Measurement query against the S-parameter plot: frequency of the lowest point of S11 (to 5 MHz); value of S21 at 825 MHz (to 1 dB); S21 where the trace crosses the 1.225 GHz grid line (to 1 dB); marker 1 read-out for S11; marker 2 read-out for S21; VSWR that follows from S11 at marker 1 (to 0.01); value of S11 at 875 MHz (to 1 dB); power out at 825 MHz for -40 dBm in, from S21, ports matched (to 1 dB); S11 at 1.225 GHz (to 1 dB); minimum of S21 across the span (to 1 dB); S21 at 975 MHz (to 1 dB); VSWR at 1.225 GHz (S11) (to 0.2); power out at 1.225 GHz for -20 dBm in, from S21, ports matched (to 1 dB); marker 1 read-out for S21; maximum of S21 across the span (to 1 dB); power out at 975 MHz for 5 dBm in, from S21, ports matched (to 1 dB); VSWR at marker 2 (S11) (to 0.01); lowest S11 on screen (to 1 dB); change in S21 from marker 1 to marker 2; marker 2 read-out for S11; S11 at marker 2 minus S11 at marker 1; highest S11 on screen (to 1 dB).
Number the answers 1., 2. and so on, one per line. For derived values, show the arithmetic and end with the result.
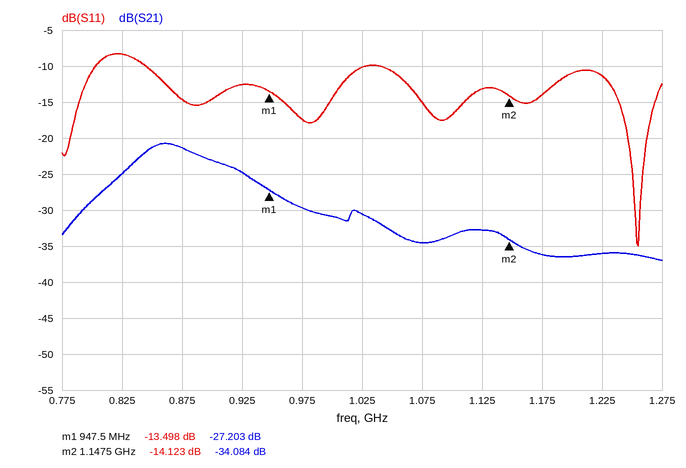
1. 1.255 GHz
2. -25 dB
3. -36 dB
4. -13.498 dB
5. -34.084 dB
6. (1 + 0.2114)/(1 − 0.2114) ≈ 1.54
7. -15 dB
8. -40 dBm + (-25 dB) = -65 dBm
9. -11 dB
10. -37 dB
11. -30 dB
12. |Γ| = 10^(-11/20) = 0.2818; VSWR = (1 + 0.2818)/(1 − 0.2818) ≈ 1.8
13. -20 dBm + (-36 dB) = -56 dBm
14. -27.203 dB
15. -21 dB
16. 5 dBm + (-30 dB) = -25 dBm
17. (1 + 0.1967)/(1 − 0.1967) ≈ 1.49
18. -35 dB
19. -34.084 − (-27.203) = -6.881 dB
20. -14.123 dB
21. -14.123 − (-13.498) = -0.625 dB
22. -8 dB
